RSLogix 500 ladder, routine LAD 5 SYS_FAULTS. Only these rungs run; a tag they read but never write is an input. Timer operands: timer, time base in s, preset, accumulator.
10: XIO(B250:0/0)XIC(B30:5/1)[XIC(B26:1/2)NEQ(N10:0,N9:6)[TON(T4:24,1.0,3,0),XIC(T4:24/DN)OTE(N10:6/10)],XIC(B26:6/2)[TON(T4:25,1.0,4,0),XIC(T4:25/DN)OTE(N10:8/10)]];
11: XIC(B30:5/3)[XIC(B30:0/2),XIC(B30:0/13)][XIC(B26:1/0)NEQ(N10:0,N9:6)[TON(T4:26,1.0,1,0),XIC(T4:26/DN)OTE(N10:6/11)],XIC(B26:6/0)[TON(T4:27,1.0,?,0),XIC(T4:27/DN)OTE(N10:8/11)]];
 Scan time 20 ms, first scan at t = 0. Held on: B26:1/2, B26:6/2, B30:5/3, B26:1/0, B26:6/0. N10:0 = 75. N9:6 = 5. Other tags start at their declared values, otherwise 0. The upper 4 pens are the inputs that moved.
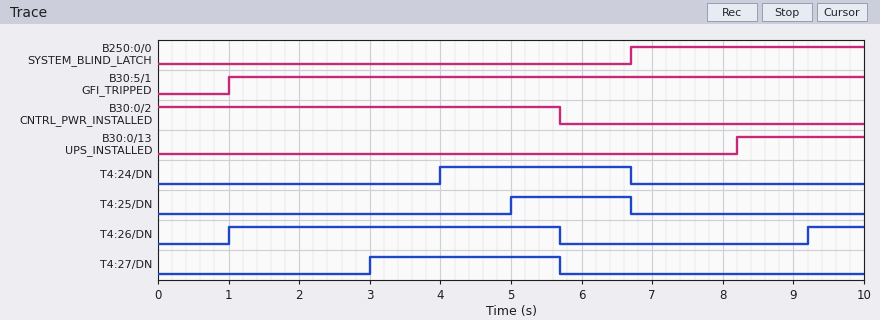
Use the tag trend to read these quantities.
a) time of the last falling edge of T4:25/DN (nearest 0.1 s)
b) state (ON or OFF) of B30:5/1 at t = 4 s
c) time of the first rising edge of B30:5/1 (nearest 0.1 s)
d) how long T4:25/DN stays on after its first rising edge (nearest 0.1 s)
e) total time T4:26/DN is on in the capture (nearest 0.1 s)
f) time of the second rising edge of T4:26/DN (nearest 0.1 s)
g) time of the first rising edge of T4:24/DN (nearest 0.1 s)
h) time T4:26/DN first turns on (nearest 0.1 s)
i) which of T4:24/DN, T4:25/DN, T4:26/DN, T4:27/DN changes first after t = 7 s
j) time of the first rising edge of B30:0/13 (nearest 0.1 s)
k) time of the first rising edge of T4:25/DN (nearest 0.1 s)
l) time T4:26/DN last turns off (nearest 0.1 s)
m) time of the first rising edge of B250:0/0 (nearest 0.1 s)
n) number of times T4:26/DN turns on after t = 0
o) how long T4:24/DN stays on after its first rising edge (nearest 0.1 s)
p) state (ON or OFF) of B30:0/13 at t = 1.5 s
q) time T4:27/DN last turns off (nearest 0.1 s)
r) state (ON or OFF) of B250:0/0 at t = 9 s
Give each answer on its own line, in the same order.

6.7 s
ON
1.0 s
1.7 s
5.5 s
9.2 s
4.0 s
1.0 s
T4:26/DN
8.2 s
5.0 s
5.7 s
6.7 s
2
2.7 s
OFF
5.7 s
ON
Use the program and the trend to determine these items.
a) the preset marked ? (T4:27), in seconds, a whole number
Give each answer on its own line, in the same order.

3 s
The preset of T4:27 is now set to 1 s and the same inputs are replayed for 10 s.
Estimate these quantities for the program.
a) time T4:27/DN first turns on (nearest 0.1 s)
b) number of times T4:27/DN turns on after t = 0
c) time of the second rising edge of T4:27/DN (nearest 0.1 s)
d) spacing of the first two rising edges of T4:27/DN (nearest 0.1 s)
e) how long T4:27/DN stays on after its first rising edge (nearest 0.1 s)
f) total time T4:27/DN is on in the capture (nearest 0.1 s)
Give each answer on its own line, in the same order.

1.0 s
2
9.2 s
8.2 s
4.7 s
5.5 s
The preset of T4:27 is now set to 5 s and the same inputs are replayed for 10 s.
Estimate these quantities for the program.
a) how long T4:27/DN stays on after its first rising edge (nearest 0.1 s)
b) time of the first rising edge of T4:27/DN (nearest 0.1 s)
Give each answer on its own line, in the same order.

0.7 s
5.0 s
